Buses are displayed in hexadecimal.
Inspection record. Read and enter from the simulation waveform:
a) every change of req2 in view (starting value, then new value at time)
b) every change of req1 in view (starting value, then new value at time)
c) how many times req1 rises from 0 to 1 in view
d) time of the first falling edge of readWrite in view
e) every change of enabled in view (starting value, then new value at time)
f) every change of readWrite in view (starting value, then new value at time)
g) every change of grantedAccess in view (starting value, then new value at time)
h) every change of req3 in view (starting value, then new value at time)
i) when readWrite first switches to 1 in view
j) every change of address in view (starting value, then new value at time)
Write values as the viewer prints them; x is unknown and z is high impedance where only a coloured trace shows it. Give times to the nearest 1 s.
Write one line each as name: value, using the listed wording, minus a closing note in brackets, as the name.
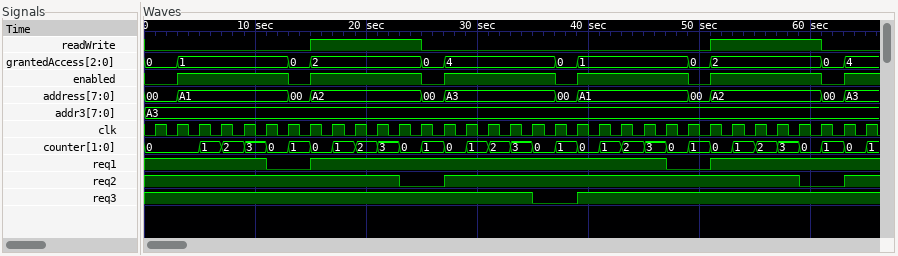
every change of req2 in view: 1, 0 at 23 s, 1 at 27 s, 0 at 59 s, 1 at 63 s
every change of req1 in view: 1, 0 at 11 s, 1 at 15 s, 0 at 47 s, 1 at 51 s
how many times req1 rises from 0 to 1 in view: 2
time of the first falling edge of readWrite in view: 25 s
every change of enabled in view: 0, 1 at 3 s, 0 at 13 s, 1 at 15 s, 0 at 25 s, 1 at 27 s, 0 at 37 s, 1 at 39 s, 0 at 49 s, 1 at 51 s, 0 at 61 s, 1 at 63 s
every change of readWrite in view: 0, 1 at 15 s, 0 at 25 s, 1 at 51 s, 0 at 61 s
every change of grantedAccess in view: 0, 1 at 3 s, 0 at 13 s, 2 at 15 s, 0 at 25 s, 4 at 27 s, 0 at 37 s, 1 at 39 s, 0 at 49 s, 2 at 51 s, 0 at 61 s, 4 at 63 s
every change of req3 in view: 1, 0 at 35 s, 1 at 39 s
when readWrite first switches to 1 in view: 15 s
every change of address in view: 00, A1 at 3 s, 00 at 13 s, A2 at 15 s, 00 at 25 s, A3 at 27 s, 00 at 37 s, A1 at 39 s, 00 at 49 s, A2 at 51 s, 00 at 61 s, A3 at 63 s
